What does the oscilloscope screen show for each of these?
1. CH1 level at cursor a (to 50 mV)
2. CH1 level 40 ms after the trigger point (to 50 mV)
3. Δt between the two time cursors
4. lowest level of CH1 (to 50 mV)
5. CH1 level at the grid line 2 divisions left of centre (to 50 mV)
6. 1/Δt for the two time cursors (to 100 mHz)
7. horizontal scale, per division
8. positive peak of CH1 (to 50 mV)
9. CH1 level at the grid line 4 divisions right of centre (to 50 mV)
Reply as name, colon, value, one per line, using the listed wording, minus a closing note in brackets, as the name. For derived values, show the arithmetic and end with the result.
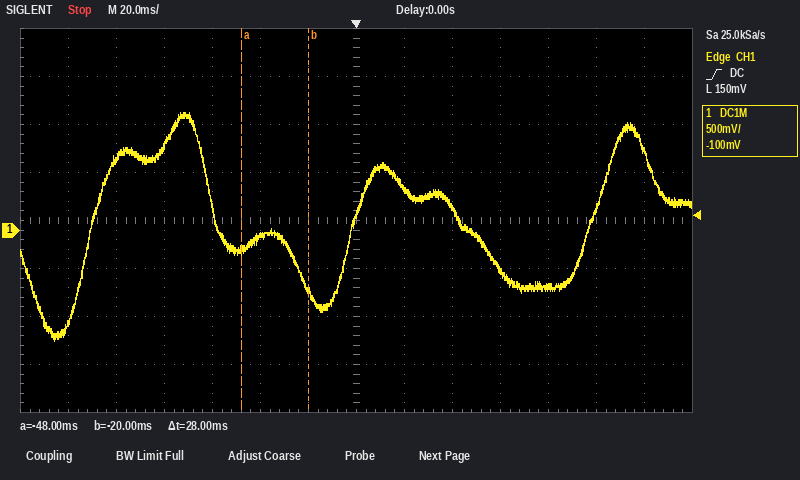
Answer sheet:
CH1 level at cursor a: -200 mV
CH1 level 40 ms after the trigger point: 250 mV
Δt between the two time cursors: 28 ms
lowest level of CH1: -1.15 V
CH1 level at the grid line 2 divisions left of centre: -50 mV
1/Δt for the two time cursors: 1 / 28 ms ≈ 35.7 Hz
horizontal scale, per division: 20 ms
positive peak of CH1: 1.20 V
CH1 level at the grid line 4 divisions right of centre: -600 mV
